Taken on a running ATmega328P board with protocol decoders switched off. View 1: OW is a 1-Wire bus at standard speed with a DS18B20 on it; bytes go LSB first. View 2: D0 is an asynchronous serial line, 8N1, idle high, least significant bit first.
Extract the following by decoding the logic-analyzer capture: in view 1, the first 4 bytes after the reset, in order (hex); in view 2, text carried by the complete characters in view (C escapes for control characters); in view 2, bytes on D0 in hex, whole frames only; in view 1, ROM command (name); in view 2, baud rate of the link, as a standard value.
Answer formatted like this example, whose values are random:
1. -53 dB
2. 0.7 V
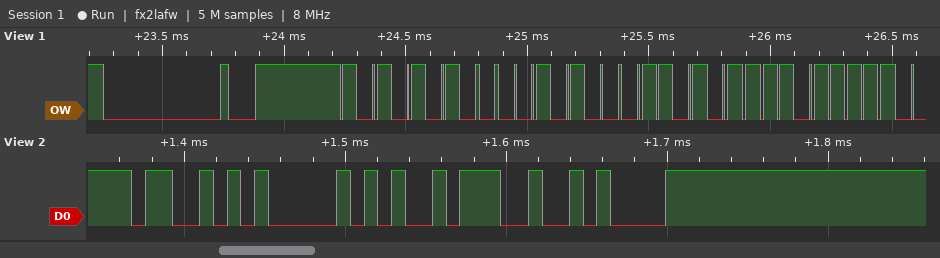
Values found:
1. 55 28 D6 FB
2. "SP:\n"
3. 53 50 3A 0A
4. Match ROM
5. 115200 baud
